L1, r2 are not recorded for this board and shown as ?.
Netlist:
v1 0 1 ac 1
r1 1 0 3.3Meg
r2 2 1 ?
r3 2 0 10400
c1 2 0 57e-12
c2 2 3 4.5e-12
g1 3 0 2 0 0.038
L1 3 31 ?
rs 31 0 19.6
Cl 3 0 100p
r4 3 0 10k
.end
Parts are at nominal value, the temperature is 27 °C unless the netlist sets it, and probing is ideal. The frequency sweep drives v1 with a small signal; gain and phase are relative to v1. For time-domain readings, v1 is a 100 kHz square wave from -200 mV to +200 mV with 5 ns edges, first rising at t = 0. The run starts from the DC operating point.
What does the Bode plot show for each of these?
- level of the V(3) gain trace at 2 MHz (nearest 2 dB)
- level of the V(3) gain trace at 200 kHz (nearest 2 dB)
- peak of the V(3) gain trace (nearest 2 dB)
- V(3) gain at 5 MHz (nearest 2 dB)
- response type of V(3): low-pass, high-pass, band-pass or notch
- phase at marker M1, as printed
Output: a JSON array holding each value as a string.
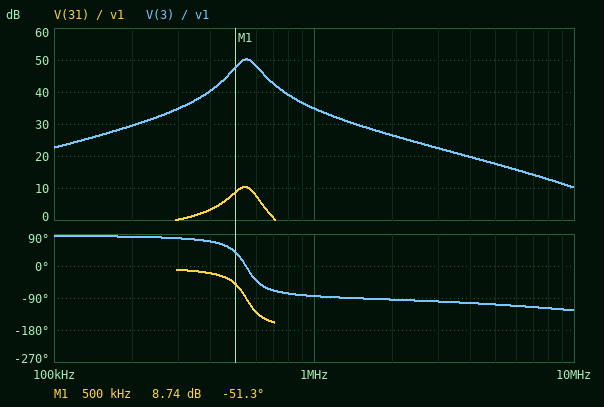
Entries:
["26 dB", "30 dB", "50 dB", "18 dB", "band-pass", "-51.3 deg"]
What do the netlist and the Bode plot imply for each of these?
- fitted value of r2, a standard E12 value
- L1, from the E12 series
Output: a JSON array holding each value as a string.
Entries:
["270 Ω", "560 µH"]
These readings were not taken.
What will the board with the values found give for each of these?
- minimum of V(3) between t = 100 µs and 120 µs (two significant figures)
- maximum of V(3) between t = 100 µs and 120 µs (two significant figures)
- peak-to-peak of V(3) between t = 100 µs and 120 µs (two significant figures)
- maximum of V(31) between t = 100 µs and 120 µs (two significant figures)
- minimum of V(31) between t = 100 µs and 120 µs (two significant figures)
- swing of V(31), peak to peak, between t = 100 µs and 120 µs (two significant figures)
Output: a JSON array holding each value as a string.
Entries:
["-25 V", "25 V", "50 V", "350 mV", "-350 mV", "710 mV"]
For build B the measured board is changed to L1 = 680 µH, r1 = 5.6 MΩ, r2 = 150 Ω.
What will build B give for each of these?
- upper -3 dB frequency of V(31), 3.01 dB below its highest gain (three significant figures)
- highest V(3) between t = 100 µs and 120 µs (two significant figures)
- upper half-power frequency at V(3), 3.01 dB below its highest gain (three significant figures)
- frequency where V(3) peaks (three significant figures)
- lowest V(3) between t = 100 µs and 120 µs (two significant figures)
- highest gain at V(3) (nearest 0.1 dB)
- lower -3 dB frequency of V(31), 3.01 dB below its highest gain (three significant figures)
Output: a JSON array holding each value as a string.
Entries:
["590 kHz", "31 V", "605 kHz", "536 kHz", "-31 V", "50.9 dB", "458 kHz"]
